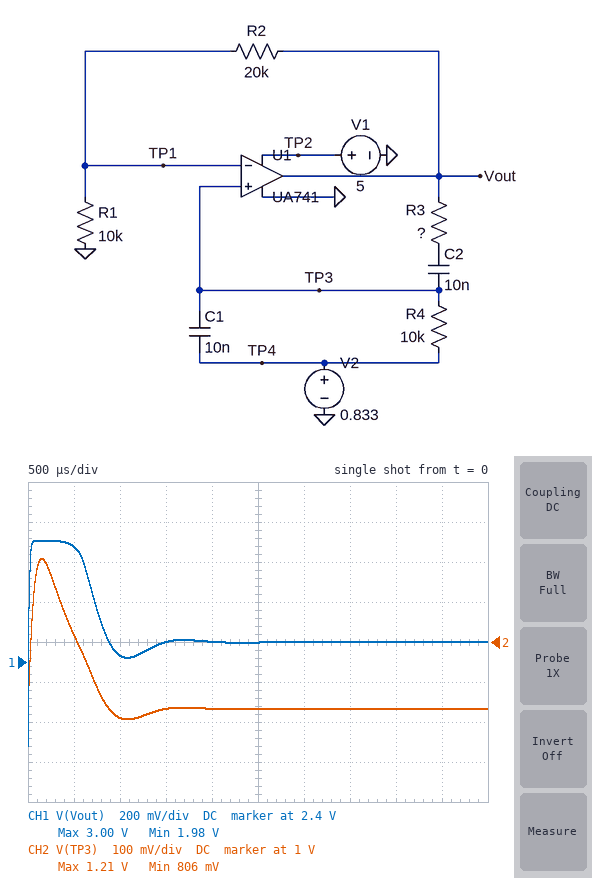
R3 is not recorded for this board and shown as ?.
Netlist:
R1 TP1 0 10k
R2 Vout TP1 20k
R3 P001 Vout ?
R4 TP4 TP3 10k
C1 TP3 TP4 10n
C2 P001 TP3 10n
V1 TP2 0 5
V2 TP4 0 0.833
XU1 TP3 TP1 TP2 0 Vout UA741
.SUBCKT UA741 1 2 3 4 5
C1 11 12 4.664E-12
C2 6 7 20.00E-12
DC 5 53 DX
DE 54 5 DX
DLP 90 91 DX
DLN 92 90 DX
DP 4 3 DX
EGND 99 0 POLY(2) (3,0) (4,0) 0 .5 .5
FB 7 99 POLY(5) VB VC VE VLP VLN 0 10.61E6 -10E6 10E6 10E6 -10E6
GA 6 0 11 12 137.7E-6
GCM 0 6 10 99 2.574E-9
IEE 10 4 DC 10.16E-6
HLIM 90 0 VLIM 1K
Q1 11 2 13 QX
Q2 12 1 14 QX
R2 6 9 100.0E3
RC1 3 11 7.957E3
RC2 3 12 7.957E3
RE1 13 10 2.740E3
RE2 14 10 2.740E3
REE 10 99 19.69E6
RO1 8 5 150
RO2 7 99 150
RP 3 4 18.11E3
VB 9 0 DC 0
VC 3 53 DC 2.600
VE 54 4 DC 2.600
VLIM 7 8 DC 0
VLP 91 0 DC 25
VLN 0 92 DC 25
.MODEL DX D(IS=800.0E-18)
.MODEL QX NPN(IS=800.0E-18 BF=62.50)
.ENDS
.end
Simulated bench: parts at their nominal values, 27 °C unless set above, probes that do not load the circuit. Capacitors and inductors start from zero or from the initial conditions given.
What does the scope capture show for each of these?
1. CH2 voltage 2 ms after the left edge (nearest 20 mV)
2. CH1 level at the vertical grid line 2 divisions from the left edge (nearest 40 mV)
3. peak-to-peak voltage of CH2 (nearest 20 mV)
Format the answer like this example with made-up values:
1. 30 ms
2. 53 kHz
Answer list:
1. 840 mV
2. 2.44 V
3. 400 mV
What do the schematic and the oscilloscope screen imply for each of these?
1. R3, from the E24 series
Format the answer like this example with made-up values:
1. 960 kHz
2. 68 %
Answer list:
1. 27 kΩ
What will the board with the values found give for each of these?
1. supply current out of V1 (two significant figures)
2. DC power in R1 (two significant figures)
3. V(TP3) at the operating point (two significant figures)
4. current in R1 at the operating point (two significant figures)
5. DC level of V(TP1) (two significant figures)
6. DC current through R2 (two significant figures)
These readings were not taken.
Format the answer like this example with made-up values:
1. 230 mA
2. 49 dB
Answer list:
1. 290 µA
2. 69 µW
3. 830 mV
4. 83 µA
5. 830 mV
6. 83 µA
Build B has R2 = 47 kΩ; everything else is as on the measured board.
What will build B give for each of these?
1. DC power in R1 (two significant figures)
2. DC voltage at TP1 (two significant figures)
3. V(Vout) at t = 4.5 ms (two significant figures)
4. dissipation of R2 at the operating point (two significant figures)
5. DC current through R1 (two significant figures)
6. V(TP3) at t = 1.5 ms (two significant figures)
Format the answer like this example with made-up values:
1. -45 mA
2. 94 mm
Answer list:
1. 28 µW
2. 530 mV
3. 3.0 V
4. 130 µW
5. 53 µA
6. 850 mV
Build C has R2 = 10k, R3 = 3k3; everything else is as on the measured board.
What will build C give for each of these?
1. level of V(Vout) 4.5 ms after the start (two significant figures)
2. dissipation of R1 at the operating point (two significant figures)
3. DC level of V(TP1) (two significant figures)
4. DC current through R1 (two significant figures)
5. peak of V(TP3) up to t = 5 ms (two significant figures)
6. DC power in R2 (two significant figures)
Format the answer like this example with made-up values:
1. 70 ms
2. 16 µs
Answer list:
1. 2.0 V
2. 99 µW
3. 1.0 V
4. 100 µA
5. 1.6 V
6. 100 µW
